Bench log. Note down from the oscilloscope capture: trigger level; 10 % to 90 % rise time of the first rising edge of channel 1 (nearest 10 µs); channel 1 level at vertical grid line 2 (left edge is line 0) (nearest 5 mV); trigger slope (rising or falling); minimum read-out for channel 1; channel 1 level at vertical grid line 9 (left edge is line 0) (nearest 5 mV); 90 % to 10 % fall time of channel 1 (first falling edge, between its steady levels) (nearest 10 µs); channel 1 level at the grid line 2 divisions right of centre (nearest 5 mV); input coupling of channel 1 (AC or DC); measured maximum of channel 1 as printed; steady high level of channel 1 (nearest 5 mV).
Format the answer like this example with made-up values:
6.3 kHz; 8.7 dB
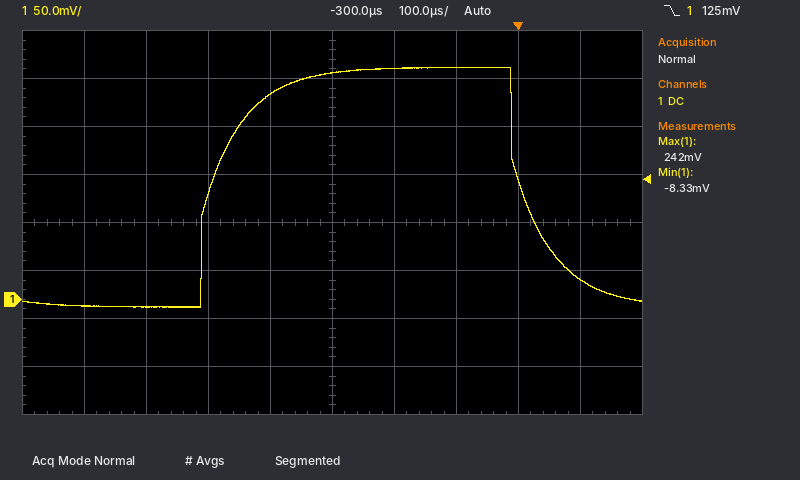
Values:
125 mV; 120 µs; -10 mV; falling; -8.33 mV; 20 mV; 120 µs; 240 mV; DC; 242 mV; 240 mV
